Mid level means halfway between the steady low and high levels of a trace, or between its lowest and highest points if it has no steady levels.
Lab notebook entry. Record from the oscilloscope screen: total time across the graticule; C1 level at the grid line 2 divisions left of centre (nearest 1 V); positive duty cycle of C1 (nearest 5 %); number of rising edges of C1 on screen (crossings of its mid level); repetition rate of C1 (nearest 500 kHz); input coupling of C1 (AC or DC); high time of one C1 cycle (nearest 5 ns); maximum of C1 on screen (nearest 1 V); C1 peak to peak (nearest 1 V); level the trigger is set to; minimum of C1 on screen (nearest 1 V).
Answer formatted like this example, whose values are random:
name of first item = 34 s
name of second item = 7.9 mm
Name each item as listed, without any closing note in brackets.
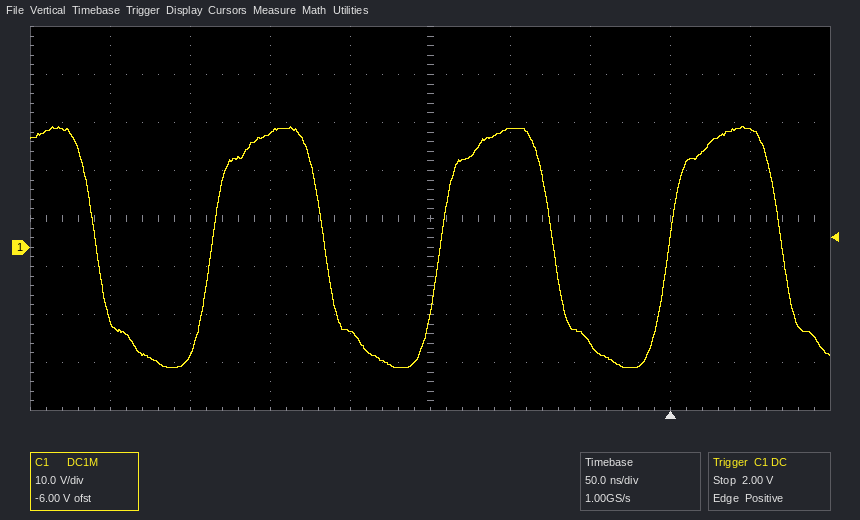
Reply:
total time across the graticule = 500 ns
C1 level at the grid line 2 divisions left of centre = 24 V
positive duty cycle of C1 = 50 %
number of rising edges of C1 on screen = 3
repetition rate of C1 = 7.0 MHz
input coupling of C1 = DC
high time of one C1 cycle = 70 ns
maximum of C1 on screen = 25 V
C1 peak to peak = 50 V
level the trigger is set to = 2.00 V
minimum of C1 on screen = -25 V
